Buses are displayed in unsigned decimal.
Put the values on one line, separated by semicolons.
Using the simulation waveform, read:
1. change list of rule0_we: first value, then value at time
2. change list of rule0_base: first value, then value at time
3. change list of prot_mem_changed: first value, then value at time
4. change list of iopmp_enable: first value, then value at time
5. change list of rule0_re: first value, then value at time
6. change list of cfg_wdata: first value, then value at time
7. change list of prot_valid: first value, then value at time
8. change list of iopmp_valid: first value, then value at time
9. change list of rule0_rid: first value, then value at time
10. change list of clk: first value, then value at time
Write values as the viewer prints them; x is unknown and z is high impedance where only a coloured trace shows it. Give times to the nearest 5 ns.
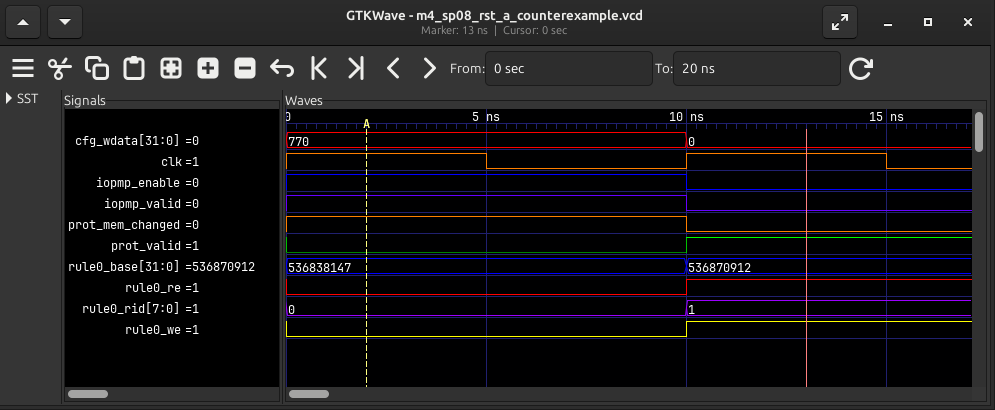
0, 1 at 10 ns; 536838147, 536870912 at 10 ns; 1, 0 at 10 ns; 1, 0 at 10 ns; 0, 1 at 10 ns; 770, 0 at 10 ns; 0, 1 at 10 ns; 1, 0 at 10 ns; 0, 1 at 10 ns; 1, 0 at 5 ns, 1 at 10 ns, 0 at 15 ns
